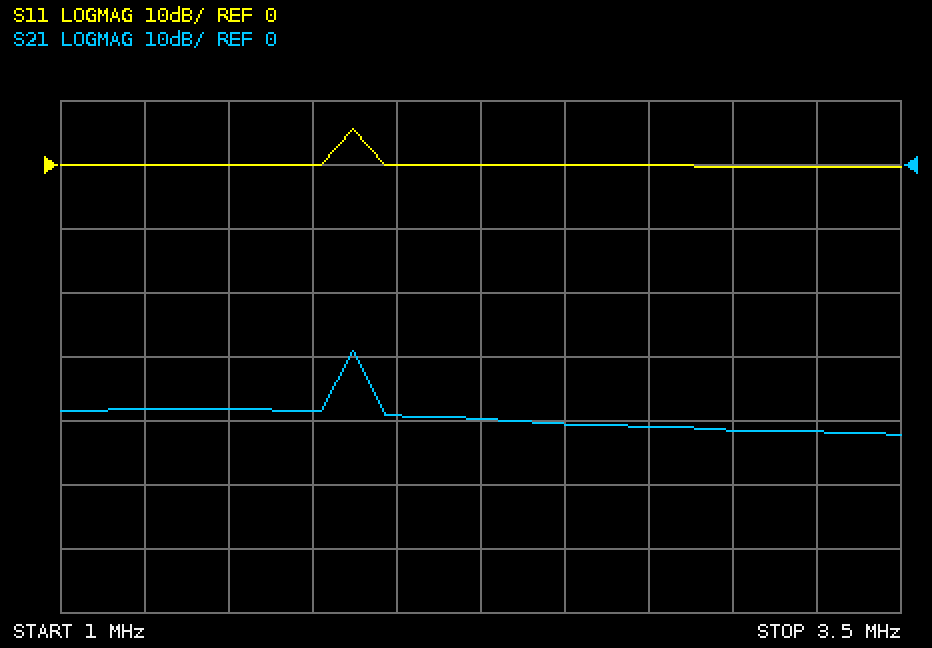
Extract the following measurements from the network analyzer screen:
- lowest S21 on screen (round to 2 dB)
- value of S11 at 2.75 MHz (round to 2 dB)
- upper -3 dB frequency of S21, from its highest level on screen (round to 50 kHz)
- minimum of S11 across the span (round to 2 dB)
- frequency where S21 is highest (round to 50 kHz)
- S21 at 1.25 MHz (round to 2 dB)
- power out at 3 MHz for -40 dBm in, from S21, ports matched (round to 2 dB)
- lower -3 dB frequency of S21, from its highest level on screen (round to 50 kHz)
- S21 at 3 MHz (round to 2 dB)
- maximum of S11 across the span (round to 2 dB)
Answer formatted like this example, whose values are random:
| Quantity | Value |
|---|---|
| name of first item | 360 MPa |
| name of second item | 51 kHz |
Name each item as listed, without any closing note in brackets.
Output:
| Quantity | Value |
|---|---|
| lowest S21 on screen | -42 dB |
| value of S11 at 2.75 MHz | 0 dB |
| upper -3 dB frequency of S21, from its highest level on screen | 1.90 MHz |
| minimum of S11 across the span | 0 dB |
| frequency where S21 is highest | 1.85 MHz |
| S21 at 1.25 MHz | -38 dB |
| power out at 3 MHz for -40 dBm in, from S21, ports matched | -82 dBm |
| lower -3 dB frequency of S21, from its highest level on screen | 1.85 MHz |
| S21 at 3 MHz | -42 dB |
| maximum of S11 across the span | 6 dB |
